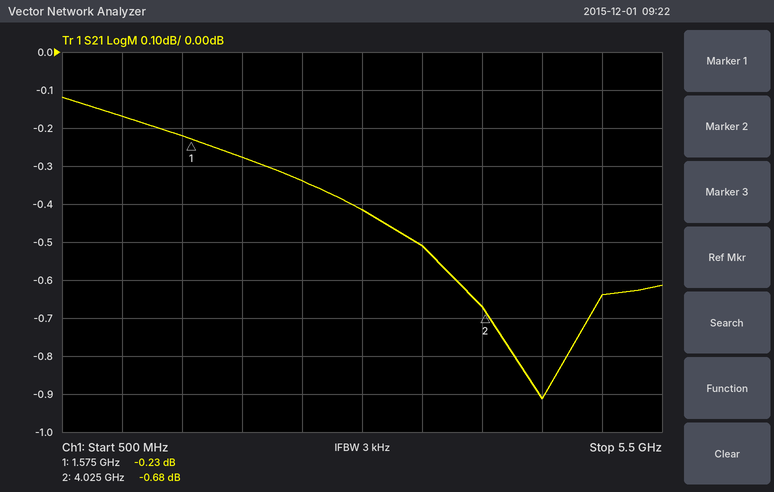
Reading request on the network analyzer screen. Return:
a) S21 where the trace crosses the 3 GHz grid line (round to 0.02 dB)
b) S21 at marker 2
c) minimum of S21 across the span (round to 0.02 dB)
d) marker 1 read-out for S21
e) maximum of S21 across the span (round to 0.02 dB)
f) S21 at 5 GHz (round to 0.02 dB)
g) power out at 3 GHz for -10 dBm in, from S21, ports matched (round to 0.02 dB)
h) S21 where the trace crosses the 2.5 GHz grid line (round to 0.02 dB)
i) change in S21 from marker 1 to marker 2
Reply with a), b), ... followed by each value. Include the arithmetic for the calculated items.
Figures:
a) -0.42 dB
b) -0.68 dB
c) -0.92 dB
d) -0.23 dB
e) -0.12 dB
f) -0.64 dB
g) -10 dBm + (-0.42 dB) = -10.42 dBm
h) -0.34 dB
i) -0.68 − (-0.23) = -0.45 dB
